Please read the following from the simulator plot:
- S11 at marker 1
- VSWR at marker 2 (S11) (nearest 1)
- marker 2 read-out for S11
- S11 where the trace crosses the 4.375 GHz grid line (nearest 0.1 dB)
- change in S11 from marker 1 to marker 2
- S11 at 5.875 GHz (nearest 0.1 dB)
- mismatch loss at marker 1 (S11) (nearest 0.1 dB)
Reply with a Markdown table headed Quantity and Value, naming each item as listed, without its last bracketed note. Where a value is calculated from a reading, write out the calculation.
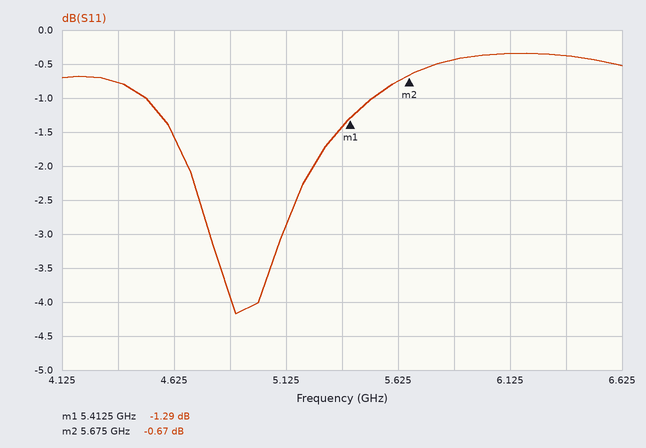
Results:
| Quantity | Value |
|---|---|
| S11 at marker 1 | -1.29 dB |
| VSWR at marker 2 (S11) | (1 + 0.9258)/(1 − 0.9258) ≈ 26 |
| marker 2 read-out for S11 | -0.67 dB |
| S11 where the trace crosses the 4.375 GHz grid line | -0.8 dB |
| change in S11 from marker 1 to marker 2 | -0.67 − (-1.29) = 0.62 dB |
| S11 at 5.875 GHz | -0.4 dB |
| mismatch loss at marker 1 (S11) | −10 log10(1 − 10^(-1.29/10)) ≈ 5.9 dB |
